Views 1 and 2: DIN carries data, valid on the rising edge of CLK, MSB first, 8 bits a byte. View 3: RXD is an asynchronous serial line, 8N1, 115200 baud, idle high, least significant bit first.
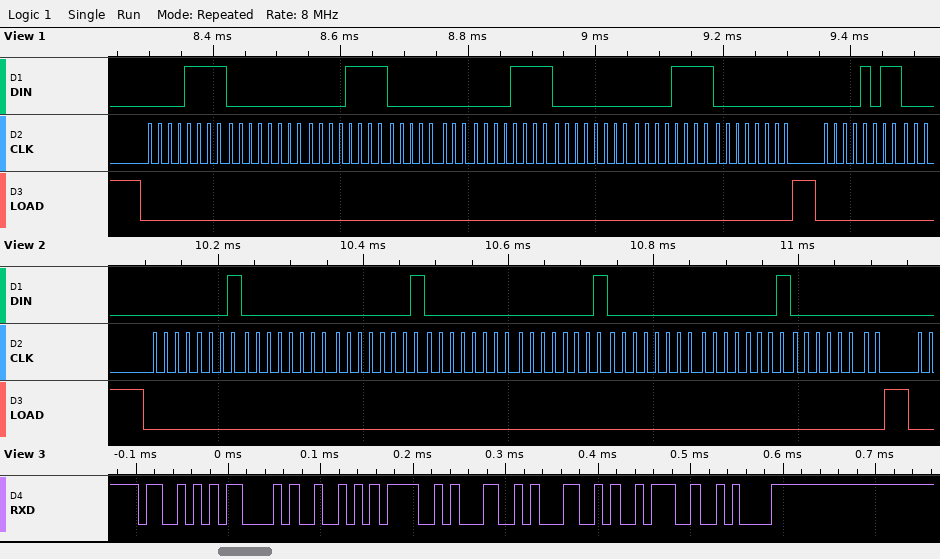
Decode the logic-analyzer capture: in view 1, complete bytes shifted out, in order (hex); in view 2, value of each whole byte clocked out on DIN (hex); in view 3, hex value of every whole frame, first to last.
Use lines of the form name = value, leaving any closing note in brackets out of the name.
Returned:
in view 1, complete bytes shifted out, in order = 0F 00 0F 00 0F 00 0F 00 0B
in view 2, value of each whole byte clocked out on DIN = 0x01 0x00 0x01 0x00 0x01 0x00 0x01 0x00
in view 3, hex value of every whole frame, first to last = 53 43 52 4F 4C 4C 3A 0A
